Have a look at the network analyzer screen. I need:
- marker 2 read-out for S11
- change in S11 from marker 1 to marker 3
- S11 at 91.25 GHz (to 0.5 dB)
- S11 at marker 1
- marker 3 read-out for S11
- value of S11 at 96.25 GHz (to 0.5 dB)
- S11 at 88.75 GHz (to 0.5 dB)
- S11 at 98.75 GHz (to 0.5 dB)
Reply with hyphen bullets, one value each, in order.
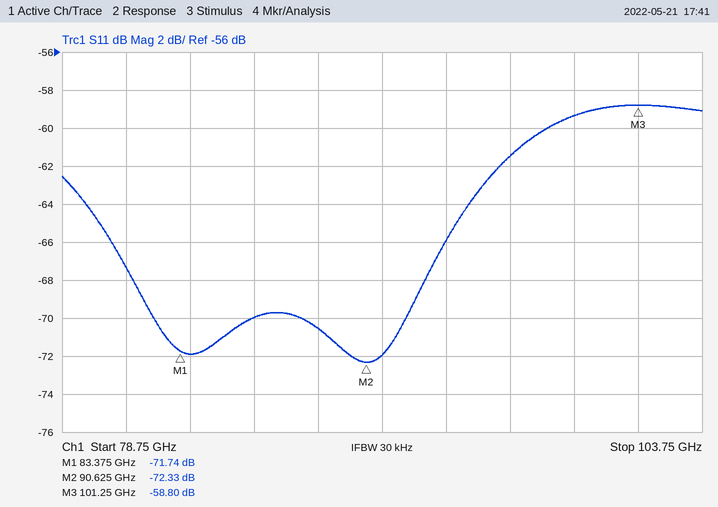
- -72.33 dB
- 12.94 dB
- -72.0 dB
- -71.74 dB
- -58.80 dB
- -61.5 dB
- -70.5 dB
- -59.5 dB
